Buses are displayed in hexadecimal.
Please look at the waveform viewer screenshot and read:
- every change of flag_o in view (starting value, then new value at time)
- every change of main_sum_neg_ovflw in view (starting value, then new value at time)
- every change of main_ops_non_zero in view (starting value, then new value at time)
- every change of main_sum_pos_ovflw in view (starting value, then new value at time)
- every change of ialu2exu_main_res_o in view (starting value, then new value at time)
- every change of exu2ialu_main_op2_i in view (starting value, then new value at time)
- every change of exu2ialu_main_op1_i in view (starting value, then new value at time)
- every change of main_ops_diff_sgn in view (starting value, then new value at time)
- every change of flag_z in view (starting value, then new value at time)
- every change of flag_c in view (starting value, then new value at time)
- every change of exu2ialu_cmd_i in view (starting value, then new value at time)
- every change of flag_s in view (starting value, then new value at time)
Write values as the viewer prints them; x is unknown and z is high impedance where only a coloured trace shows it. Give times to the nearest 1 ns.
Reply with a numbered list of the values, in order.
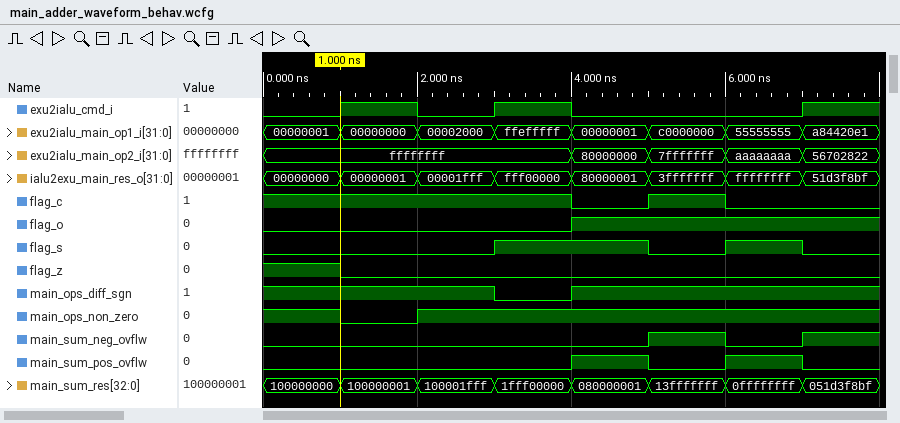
1. 0, 1 at 4 ns
2. 0, 1 at 5 ns, 0 at 6 ns, 1 at 7 ns
3. 1, 0 at 1 ns, 1 at 2 ns
4. 0, 1 at 4 ns, 0 at 5 ns, 1 at 6 ns, 0 at 7 ns
5. 00000000, 00000001 at 1 ns, 00001fff at 2 ns, fff00000 at 3 ns, 80000001 at 4 ns, 3fffffff at 5 ns, ffffffff at 6 ns, 51d3f8bf at 7 ns
6. ffffffff, 80000000 at 4 ns, 7fffffff at 5 ns, aaaaaaaa at 6 ns, 56702822 at 7 ns
7. 00000001, 00000000 at 1 ns, 00002000 at 2 ns, ffefffff at 3 ns, 00000001 at 4 ns, c0000000 at 5 ns, 55555555 at 6 ns, a84420e1 at 7 ns
8. 1, 0 at 3 ns, 1 at 4 ns
9. 1, 0 at 1 ns
10. 1, 0 at 4 ns, 1 at 5 ns, 0 at 6 ns
11. 0, 1 at 1 ns, 0 at 2 ns, 1 at 3 ns, 0 at 4 ns, 1 at 7 ns
12. 0, 1 at 3 ns, 0 at 5 ns, 1 at 6 ns, 0 at 7 ns
